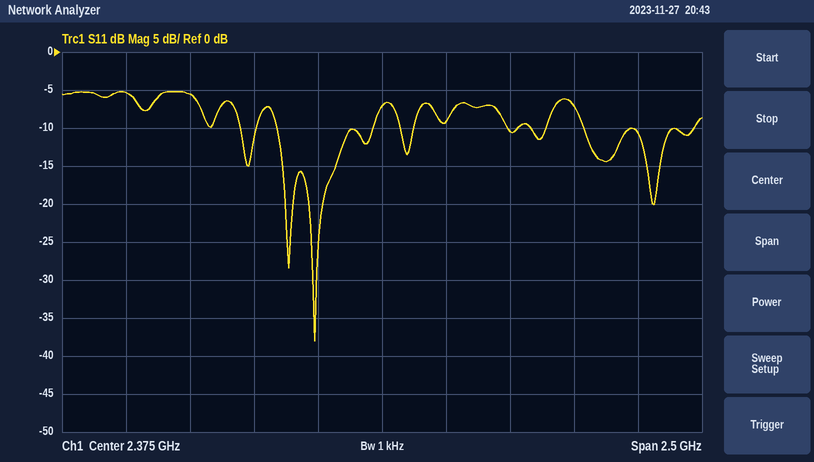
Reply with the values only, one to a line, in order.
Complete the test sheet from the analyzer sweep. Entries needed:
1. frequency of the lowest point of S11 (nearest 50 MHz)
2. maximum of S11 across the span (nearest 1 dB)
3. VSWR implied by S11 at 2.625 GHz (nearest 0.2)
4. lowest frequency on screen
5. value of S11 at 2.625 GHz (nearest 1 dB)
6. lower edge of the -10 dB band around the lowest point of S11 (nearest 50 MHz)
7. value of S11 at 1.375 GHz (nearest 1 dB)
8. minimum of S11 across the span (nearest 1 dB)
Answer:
2.10 GHz
-5 dB
2.0
1.125 GHz
-9 dB
1.95 GHz
-5 dB
-38 dB
